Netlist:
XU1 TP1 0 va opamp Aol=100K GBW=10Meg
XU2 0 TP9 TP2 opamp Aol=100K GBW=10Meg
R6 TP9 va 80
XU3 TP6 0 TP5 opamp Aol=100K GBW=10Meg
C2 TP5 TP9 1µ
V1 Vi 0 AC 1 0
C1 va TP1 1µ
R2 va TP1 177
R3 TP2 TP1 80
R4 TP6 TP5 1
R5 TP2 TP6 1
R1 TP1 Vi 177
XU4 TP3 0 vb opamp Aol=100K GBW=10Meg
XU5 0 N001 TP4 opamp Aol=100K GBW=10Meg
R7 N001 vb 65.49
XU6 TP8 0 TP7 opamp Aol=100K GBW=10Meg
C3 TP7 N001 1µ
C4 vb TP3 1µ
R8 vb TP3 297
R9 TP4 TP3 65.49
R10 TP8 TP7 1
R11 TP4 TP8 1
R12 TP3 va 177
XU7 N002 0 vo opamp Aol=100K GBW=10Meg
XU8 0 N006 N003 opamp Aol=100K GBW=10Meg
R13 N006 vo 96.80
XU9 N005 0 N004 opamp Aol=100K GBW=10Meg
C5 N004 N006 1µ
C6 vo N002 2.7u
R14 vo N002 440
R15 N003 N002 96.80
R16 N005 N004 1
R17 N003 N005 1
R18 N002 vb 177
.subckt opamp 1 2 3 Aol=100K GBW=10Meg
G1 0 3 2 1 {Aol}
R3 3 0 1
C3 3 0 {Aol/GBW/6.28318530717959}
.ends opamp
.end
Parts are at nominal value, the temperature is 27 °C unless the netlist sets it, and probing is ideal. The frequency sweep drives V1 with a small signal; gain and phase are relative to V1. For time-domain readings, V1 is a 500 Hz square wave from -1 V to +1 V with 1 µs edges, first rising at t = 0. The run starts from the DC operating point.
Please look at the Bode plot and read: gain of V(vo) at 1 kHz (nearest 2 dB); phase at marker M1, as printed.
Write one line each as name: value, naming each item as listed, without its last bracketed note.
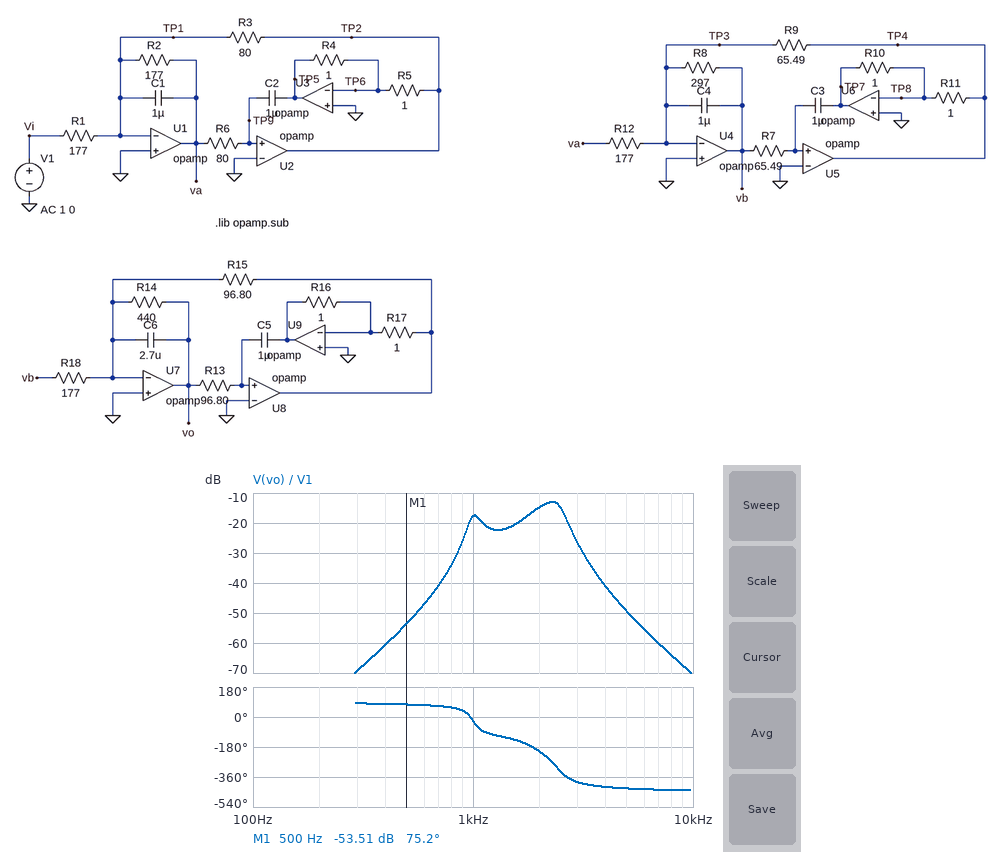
gain of V(vo) at 1 kHz: -18 dB
phase at marker M1, as printed: 75.2 deg
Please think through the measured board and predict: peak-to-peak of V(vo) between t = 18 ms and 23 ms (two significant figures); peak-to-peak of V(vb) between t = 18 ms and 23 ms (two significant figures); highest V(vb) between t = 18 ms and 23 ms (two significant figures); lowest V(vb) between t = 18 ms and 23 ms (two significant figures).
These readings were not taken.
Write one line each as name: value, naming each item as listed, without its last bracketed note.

peak-to-peak of V(vo) between t = 18 ms and 23 ms: 160 mV
peak-to-peak of V(vb) between t = 18 ms and 23 ms: 740 mV
highest V(vb) between t = 18 ms and 23 ms: 370 mV
lowest V(vb) between t = 18 ms and 23 ms: -370 mV
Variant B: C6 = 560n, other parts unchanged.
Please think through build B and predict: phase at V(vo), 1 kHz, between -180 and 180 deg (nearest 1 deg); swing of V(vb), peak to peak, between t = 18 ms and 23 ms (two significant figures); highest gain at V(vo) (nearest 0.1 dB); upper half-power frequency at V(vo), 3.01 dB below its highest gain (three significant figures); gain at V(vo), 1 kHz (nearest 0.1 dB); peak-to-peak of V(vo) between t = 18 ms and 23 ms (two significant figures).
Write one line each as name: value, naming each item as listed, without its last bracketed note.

phase at V(vo), 1 kHz, between -180 and 180 deg: 57 deg
swing of V(vb), peak to peak, between t = 18 ms and 23 ms: 740 mV
highest gain at V(vo): 9.5 dB
upper half-power frequency at V(vo), 3.01 dB below its highest gain: 2.50 kHz
gain at V(vo), 1 kHz: -33.2 dB
peak-to-peak of V(vo) between t = 18 ms and 23 ms: 1.2 V
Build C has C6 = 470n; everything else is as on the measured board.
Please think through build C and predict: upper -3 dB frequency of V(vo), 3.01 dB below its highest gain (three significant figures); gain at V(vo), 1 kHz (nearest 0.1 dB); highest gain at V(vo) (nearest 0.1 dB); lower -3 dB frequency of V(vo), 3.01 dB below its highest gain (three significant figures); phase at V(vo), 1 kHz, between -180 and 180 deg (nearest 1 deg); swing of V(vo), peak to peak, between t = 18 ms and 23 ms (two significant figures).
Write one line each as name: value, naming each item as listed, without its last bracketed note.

upper -3 dB frequency of V(vo), 3.01 dB below its highest gain: 2.57 kHz
gain at V(vo), 1 kHz: -33.5 dB
highest gain at V(vo): 10.1 dB
lower -3 dB frequency of V(vo), 3.01 dB below its highest gain: 2.16 kHz
phase at V(vo), 1 kHz, between -180 and 180 deg: 58 deg
swing of V(vo), peak to peak, between t = 18 ms and 23 ms: 1.5 V
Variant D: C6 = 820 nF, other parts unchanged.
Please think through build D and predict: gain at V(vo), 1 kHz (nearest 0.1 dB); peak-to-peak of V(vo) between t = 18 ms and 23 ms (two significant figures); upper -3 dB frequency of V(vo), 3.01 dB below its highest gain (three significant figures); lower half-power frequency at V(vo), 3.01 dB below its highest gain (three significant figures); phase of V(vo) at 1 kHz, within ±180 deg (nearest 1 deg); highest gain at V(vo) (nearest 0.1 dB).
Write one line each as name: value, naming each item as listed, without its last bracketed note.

gain at V(vo), 1 kHz: -32.1 dB
peak-to-peak of V(vo) between t = 18 ms and 23 ms: 720 mV
upper -3 dB frequency of V(vo), 3.01 dB below its highest gain: 2.45 kHz
lower half-power frequency at V(vo), 3.01 dB below its highest gain: 1.76 kHz
phase of V(vo) at 1 kHz, within ±180 deg: 56 deg
highest gain at V(vo): 4.1 dB
